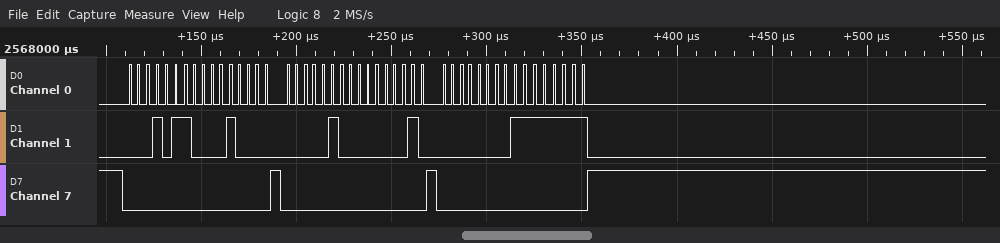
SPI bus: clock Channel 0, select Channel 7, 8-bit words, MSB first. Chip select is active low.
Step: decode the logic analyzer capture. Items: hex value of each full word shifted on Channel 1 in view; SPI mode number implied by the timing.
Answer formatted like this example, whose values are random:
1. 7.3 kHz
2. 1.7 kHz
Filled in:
1. 16, 10, 04, 02, 00, FF
2. 1
